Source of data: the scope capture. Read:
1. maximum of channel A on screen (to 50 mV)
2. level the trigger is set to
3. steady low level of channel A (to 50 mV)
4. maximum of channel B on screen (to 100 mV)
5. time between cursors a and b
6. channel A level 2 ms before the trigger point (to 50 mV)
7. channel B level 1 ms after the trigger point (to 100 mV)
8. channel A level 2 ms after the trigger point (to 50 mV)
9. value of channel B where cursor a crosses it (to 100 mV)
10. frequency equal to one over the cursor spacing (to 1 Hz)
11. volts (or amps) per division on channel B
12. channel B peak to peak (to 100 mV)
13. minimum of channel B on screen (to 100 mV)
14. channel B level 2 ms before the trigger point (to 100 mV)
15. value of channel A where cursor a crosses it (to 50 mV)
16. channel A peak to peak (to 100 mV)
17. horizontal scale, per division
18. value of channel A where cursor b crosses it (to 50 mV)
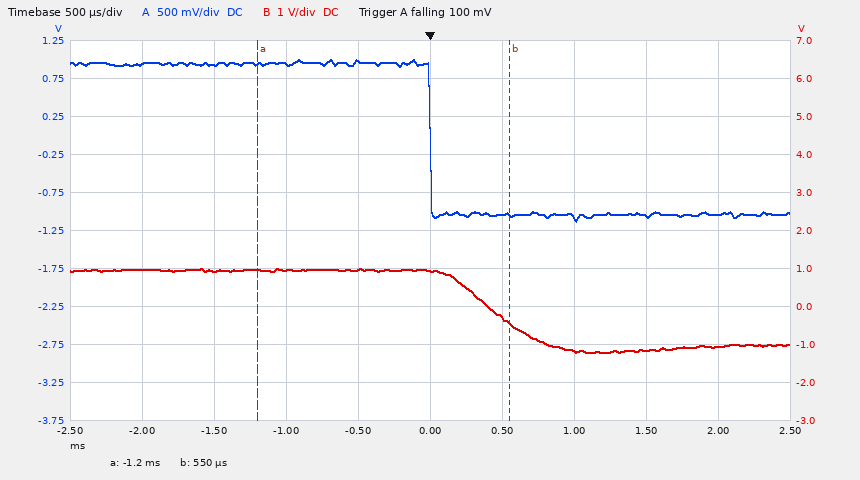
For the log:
1.00 V
100 mV
-1.05 V
1.0 V
1.75 ms
950 mV
-1.2 V
-1.05 V
1.0 V
571 Hz
1 V
2.2 V
-1.2 V
1.0 V
950 mV
2.10 V
500 µs
-1.05 V
